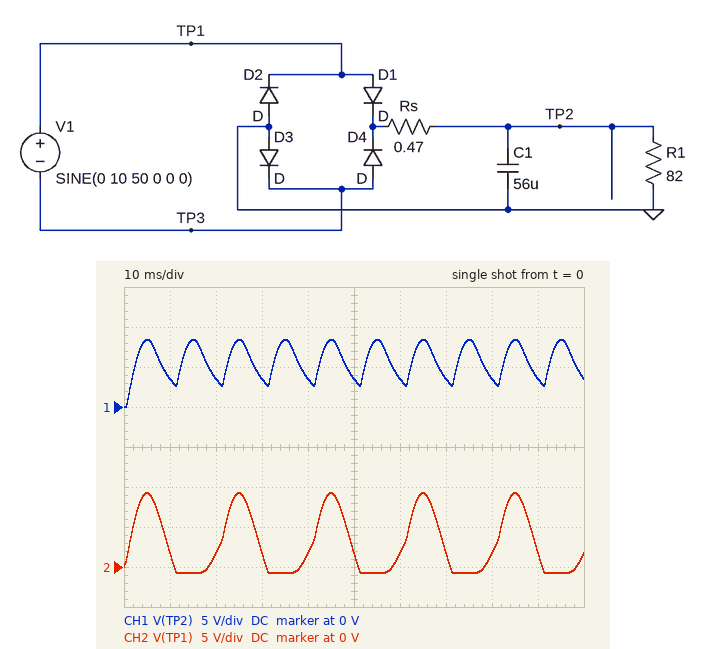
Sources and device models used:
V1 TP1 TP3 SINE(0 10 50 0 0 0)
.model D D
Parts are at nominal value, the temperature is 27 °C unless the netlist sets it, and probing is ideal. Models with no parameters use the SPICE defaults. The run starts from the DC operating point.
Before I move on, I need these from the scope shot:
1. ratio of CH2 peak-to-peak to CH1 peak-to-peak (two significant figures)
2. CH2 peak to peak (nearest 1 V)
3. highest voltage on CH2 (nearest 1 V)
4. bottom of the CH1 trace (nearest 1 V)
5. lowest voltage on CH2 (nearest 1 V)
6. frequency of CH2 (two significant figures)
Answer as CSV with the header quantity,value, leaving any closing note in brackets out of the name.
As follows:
quantity,value
ratio of CH2 peak-to-peak to CH1 peak-to-peak,1.2
CH2 peak to peak,10 V
highest voltage on CH2,9 V
bottom of the CH1 trace,0 V
lowest voltage on CH2,-1 V
frequency of CH2,50 Hz
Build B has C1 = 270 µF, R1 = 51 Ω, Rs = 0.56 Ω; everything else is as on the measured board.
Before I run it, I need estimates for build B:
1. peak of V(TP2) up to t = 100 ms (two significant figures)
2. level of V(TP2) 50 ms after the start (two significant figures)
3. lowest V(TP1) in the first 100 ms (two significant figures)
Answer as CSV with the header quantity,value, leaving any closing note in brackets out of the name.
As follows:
quantity,value
peak of V(TP2) up to t = 100 ms,8.3 V
level of V(TP2) 50 ms after the start,6.0 V
lowest V(TP1) in the first 100 ms,-820 mV
